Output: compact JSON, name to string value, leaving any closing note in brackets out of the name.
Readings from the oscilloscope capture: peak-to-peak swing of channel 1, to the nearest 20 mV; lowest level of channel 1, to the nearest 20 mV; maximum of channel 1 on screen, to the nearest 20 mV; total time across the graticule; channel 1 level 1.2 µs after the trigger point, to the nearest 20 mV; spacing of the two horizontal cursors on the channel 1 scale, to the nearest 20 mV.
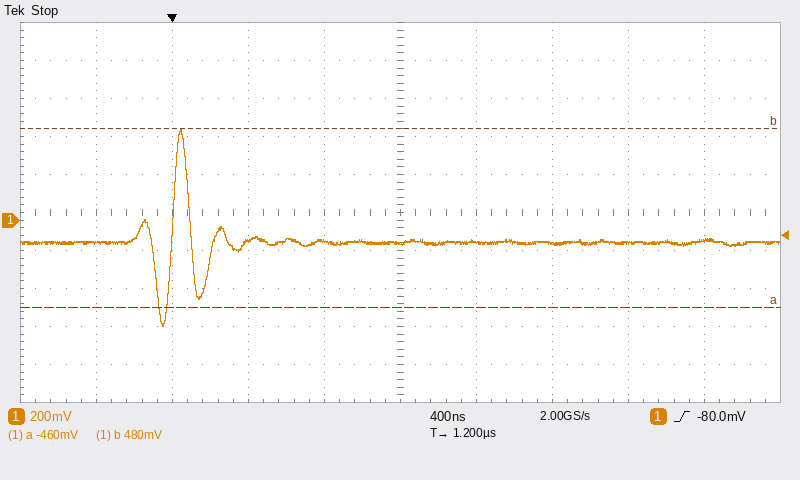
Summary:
{"peak-to-peak swing of channel 1, to the nearest 20 mV": "1.04 V", "lowest level of channel 1, to the nearest 20 mV": "-560 mV", "maximum of channel 1 on screen, to the nearest 20 mV": "480 mV", "total time across the graticule": "4 µs", "channel 1 level 1.2 µs after the trigger point, to the nearest 20 mV": "-120 mV", "spacing of the two horizontal cursors on the channel 1 scale, to the nearest 20 mV": "940 mV"}
